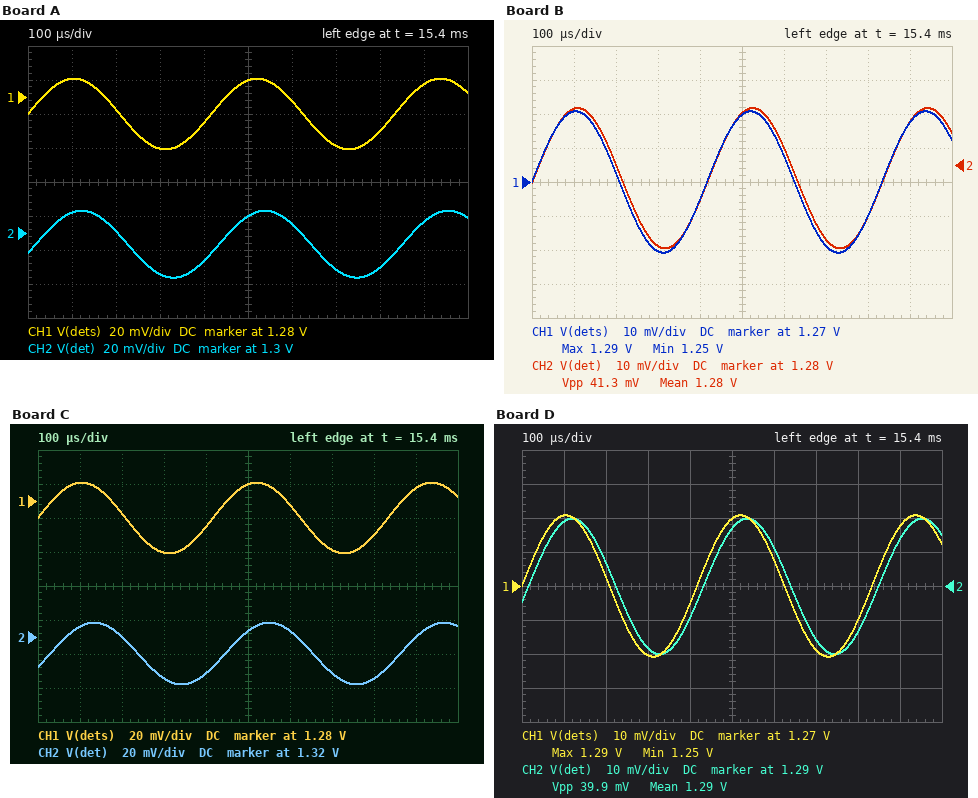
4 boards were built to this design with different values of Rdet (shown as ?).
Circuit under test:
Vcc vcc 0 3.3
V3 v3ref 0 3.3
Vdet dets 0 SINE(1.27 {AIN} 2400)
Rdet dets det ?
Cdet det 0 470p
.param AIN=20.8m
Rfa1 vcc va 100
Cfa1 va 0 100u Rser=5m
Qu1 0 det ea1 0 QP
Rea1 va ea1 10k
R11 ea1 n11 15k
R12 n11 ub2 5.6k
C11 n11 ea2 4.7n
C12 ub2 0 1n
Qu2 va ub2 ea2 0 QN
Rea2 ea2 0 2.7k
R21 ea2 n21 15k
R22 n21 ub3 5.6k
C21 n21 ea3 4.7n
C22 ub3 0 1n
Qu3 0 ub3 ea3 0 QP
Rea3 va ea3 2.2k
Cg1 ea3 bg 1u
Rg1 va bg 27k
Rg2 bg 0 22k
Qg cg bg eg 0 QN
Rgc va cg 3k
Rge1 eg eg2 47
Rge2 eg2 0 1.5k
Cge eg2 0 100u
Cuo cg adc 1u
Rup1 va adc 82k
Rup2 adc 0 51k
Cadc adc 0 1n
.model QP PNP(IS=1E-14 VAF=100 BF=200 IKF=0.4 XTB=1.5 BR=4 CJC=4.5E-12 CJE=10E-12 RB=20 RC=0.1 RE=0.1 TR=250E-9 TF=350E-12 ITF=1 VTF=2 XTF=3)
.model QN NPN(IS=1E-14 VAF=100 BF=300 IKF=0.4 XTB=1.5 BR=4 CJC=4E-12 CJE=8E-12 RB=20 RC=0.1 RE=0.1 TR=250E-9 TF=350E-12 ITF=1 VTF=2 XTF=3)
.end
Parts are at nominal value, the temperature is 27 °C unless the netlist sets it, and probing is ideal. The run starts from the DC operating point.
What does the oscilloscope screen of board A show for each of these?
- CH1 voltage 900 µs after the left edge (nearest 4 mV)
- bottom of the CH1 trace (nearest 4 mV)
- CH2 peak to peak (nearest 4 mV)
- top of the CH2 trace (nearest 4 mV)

1.288 V
1.248 V
40 mV
1.312 V
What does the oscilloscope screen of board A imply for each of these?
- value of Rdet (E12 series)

39 kΩ
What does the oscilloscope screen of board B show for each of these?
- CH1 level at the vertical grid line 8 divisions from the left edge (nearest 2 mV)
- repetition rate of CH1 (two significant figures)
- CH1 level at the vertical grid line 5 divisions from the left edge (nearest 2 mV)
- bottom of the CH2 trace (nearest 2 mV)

1.260 V
2.4 kHz
1.290 V
1.256 V
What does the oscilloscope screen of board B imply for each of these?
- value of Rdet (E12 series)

10 kΩ
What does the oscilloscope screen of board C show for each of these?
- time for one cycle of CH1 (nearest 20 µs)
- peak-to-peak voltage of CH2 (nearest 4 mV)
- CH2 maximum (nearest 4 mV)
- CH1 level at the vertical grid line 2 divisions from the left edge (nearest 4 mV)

420 µs
36 mV
1.328 V
1.272 V
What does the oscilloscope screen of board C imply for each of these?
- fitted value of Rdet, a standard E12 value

68 kΩ
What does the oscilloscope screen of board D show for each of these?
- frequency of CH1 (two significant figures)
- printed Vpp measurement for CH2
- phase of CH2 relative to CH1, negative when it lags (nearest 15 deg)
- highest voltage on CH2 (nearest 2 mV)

2.4 kHz
39.9 mV
-15 deg
1.310 V
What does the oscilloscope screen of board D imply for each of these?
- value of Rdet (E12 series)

33 kΩ
